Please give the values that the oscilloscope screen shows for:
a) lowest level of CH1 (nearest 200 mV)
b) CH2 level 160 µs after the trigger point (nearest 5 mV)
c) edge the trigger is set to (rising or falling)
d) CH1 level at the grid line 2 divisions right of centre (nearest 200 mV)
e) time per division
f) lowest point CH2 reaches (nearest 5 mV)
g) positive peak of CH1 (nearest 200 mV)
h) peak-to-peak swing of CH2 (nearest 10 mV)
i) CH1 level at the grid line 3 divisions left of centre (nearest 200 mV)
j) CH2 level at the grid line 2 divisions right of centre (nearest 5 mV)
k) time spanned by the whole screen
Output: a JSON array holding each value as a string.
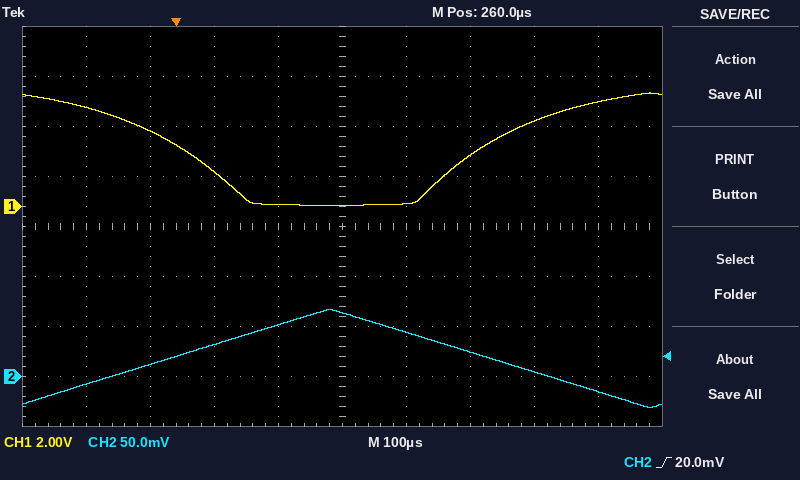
["0.0 V", "50 mV", "rising", "2.0 V", "100 µs", "-30 mV", "4.6 V", "100 mV", "3.0 V", "25 mV", "1 ms"]
